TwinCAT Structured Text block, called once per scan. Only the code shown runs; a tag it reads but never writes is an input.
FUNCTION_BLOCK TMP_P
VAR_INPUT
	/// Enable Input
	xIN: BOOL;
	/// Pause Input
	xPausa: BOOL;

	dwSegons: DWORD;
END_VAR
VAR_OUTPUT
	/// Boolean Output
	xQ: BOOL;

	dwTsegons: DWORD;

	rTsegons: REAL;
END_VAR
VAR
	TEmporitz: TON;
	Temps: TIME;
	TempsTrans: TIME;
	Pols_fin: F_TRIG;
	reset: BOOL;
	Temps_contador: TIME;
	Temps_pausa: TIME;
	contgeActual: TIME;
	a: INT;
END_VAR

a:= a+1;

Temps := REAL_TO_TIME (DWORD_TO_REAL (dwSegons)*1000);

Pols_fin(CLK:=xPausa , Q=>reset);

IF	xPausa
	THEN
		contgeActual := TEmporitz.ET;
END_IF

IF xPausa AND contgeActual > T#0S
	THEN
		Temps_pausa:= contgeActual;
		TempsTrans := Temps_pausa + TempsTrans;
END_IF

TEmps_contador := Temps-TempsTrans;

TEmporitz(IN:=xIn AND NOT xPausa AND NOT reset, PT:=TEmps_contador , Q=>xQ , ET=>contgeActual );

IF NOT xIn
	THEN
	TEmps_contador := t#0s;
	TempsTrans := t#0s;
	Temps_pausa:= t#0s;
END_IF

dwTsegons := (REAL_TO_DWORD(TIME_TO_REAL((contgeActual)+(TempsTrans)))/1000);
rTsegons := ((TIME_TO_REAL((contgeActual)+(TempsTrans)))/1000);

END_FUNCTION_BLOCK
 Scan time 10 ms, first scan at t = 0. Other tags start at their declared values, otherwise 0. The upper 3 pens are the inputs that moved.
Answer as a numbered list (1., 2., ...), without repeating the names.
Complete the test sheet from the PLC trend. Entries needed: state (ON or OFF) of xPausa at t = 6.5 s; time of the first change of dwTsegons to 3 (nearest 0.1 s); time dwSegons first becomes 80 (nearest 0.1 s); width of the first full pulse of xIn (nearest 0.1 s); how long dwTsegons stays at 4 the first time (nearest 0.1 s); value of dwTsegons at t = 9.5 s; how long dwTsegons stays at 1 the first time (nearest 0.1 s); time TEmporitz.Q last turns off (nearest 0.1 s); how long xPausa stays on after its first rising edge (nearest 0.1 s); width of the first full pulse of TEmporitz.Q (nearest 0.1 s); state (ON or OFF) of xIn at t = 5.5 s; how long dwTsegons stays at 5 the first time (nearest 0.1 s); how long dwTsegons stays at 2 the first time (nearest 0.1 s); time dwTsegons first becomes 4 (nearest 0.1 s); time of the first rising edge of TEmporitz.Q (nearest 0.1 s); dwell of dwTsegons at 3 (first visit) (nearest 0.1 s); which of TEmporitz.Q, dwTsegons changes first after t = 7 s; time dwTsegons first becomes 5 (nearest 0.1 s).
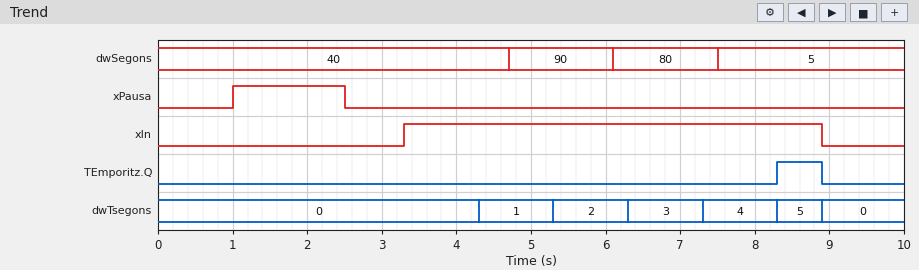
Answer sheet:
1. OFF
2. 6.3 s
3. 6.1 s
4. 5.6 s
5. 1.0 s
6. 0
7. 1.0 s
8. 8.9 s
9. 1.5 s
10. 0.6 s
11. ON
12. 0.6 s
13. 1.0 s
14. 7.3 s
15. 8.3 s
16. 1.0 s
17. dwTsegons
18. 8.3 s
